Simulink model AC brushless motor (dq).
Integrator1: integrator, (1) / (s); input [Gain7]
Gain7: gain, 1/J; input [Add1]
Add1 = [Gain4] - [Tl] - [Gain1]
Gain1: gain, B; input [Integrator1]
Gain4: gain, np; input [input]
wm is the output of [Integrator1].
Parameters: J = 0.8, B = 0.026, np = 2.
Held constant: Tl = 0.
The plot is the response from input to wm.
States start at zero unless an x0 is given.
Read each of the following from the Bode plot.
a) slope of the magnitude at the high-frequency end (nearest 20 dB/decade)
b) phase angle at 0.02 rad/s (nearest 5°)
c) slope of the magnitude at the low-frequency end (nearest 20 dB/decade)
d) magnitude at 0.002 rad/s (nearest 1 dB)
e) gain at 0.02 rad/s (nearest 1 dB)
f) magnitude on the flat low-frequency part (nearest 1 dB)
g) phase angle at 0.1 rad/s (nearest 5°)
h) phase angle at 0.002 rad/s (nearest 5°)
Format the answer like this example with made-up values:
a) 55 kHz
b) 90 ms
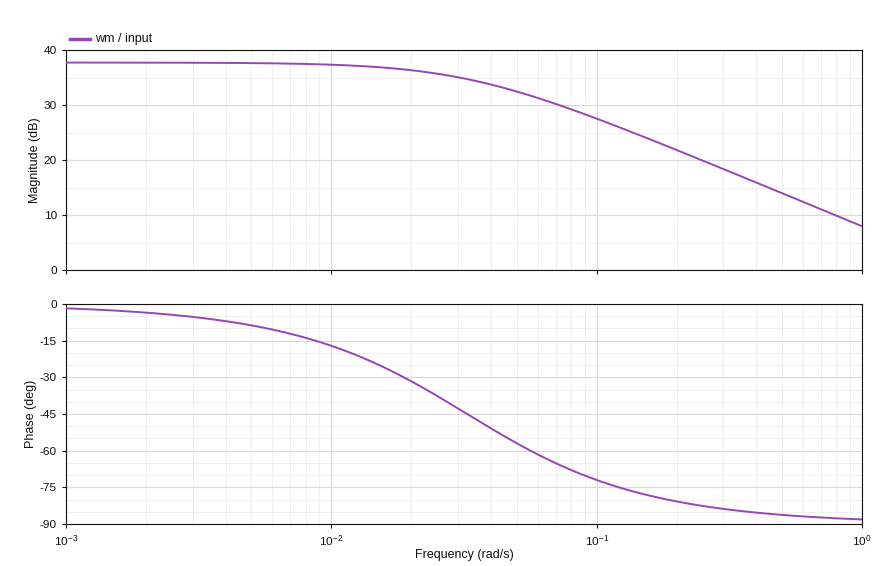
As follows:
a) -20 dB/decade
b) -30°
c) 0 dB/decade
d) 38 dB
e) 36 dB
f) 38 dB
g) -70°
h) -5°
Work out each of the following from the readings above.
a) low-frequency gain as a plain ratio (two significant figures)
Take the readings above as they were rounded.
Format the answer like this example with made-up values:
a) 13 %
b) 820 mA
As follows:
a) 79
